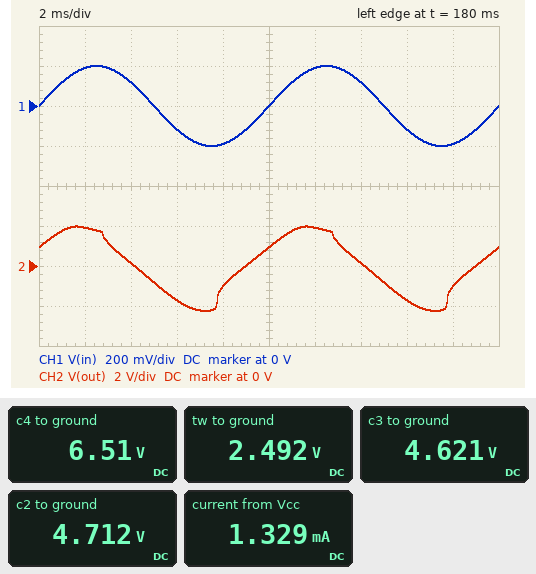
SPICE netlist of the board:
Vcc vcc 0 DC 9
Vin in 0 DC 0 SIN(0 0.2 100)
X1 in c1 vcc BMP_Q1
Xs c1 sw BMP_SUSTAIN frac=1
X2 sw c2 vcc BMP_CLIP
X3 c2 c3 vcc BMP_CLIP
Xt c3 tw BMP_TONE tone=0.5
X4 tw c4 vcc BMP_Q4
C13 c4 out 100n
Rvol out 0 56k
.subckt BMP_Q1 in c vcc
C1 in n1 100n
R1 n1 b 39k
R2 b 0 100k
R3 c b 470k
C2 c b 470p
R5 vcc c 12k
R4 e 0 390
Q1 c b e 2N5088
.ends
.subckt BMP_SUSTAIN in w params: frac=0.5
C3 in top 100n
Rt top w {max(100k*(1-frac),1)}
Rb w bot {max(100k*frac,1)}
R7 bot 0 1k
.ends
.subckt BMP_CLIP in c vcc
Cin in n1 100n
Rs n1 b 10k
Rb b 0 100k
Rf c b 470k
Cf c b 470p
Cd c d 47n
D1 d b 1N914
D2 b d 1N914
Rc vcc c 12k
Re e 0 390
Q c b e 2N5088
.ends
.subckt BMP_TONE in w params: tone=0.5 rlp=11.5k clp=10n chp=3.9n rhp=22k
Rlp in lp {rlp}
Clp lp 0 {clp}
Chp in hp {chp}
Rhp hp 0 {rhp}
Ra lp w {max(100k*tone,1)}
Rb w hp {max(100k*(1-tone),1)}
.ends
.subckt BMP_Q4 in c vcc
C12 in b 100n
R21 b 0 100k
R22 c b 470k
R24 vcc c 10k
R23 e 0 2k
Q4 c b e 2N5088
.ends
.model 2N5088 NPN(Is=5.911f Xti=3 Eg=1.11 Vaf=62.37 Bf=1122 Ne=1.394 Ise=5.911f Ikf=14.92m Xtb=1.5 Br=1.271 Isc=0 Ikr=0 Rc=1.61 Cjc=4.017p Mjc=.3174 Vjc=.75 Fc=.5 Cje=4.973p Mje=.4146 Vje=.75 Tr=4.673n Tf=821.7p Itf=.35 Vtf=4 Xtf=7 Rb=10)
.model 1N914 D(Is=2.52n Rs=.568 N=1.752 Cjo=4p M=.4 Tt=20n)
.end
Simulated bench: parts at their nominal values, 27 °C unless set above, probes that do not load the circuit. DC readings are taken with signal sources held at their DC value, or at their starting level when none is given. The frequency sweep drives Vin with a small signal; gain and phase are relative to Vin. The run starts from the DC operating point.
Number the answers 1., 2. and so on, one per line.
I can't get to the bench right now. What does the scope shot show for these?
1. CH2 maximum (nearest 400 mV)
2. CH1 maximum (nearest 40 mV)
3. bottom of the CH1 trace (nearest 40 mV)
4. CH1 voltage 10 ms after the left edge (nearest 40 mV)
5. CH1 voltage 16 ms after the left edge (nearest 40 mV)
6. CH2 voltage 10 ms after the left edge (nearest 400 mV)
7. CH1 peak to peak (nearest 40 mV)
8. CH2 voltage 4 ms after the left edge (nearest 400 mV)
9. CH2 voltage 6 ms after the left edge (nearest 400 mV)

1. 2.0 V
2. 200 mV
3. -200 mV
4. 0 V
5. -120 mV
6. 800 mV
7. 400 mV
8. 0 V
9. -1.6 V
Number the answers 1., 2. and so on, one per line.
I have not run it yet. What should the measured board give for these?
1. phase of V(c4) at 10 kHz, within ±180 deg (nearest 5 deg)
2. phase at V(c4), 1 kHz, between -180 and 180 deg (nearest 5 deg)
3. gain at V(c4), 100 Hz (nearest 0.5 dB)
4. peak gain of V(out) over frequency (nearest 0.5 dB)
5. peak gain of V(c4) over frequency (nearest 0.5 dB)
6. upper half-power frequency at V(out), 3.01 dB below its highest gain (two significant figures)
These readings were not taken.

1. 140 deg
2. -90 deg
3. 55.5 dB
4. 58.0 dB
5. 58.0 dB
6. 700 Hz
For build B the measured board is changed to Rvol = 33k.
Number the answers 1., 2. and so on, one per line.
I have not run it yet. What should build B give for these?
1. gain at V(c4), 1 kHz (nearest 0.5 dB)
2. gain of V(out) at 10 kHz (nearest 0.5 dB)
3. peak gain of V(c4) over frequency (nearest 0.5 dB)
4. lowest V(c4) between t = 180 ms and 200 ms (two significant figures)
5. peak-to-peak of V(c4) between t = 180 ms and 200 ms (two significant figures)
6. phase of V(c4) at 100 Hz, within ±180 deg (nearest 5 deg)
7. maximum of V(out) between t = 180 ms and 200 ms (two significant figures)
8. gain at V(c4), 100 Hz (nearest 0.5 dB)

1. 51.0 dB
2. 15.5 dB
3. 57.0 dB
4. 4.0 V
5. 4.4 V
6. 85 deg
7. 1.7 V
8. 55.0 dB
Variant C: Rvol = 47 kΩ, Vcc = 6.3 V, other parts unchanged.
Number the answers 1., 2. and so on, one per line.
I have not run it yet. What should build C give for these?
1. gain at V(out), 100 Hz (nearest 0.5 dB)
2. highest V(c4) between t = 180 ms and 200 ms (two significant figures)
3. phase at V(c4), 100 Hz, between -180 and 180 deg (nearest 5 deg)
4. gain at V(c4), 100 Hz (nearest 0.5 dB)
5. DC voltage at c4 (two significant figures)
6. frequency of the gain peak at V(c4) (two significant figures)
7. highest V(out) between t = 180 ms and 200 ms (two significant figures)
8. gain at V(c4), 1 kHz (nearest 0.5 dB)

1. 52.5 dB
2. 6.0 V
3. 80 deg
4. 53.0 dB
5. 5.0 V
6. 250 Hz
7. 1.2 V
8. 49.0 dB
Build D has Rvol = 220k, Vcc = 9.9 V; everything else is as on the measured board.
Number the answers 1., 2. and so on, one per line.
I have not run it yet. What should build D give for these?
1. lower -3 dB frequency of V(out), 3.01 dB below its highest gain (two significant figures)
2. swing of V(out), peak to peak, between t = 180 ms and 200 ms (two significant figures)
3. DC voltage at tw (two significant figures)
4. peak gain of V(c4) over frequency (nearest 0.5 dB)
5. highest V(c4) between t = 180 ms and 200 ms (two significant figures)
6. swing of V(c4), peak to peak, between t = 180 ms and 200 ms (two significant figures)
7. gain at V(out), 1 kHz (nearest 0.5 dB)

1. 96 Hz
2. 5.3 V
3. 2.6 V
4. 59.0 dB
5. 9.6 V
6. 5.4 V
7. 53.0 dB
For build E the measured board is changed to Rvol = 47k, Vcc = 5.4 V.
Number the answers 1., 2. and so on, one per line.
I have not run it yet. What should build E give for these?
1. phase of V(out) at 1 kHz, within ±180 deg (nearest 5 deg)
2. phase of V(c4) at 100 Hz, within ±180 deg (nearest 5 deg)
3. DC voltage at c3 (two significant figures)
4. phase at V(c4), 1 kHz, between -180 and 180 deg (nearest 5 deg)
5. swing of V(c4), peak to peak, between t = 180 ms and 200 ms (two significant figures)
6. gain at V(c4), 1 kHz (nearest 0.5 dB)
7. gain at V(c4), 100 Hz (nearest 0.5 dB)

1. -80 deg
2. 80 deg
3. 3.8 V
4. -85 deg
5. 2.0 V
6. 47.0 dB
7. 50.5 dB
